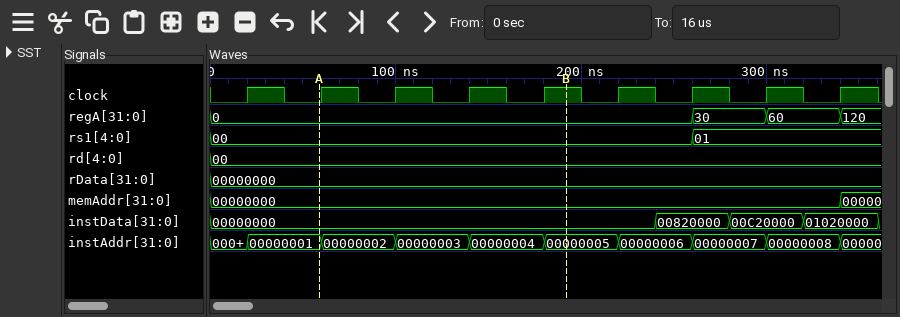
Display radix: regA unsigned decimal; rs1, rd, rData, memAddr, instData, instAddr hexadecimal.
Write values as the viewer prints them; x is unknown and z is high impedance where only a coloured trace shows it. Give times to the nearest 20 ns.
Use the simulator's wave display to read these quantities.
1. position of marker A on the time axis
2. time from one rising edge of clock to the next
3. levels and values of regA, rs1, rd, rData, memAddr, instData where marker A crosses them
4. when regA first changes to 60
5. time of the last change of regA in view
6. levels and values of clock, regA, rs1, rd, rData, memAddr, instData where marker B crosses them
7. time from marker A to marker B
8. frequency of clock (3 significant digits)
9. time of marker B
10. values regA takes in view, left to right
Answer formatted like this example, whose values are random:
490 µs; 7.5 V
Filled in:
60 ns; 40 ns; regA=0, rs1=00, rd=00, rData=00000000, memAddr=00000000, instData=00000000; 300 ns; 340 ns; clock=1, regA=0, rs1=00, rd=00, rData=00000000, memAddr=00000000, instData=00000000; 140 ns; 25.0 MHz; 200 ns; 0, 30, 60, 120
